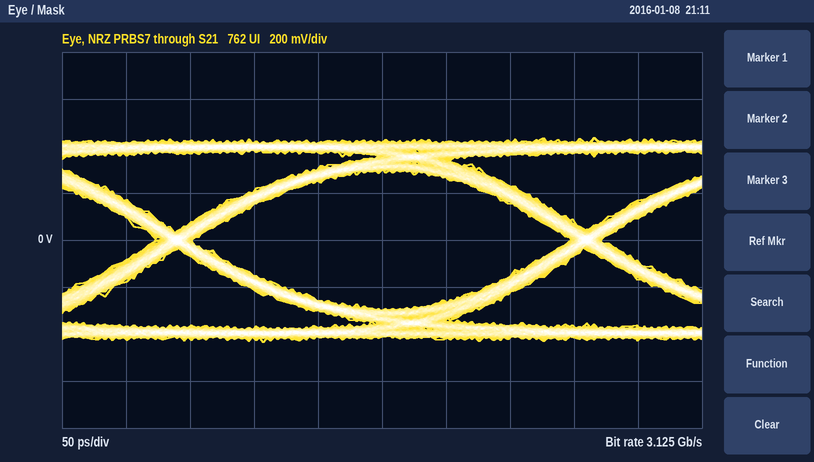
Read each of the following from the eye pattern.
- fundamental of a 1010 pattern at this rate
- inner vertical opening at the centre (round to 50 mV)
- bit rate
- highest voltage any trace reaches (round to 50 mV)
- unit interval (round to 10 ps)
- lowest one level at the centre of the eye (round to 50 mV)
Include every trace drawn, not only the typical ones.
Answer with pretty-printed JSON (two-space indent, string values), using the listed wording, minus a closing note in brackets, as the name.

{
  "fundamental of a 1010 pattern at this rate": "1.5625 GHz",
  "inner vertical opening at the centre": "600 mV",
  "bit rate": "3.125 Gb/s",
  "highest voltage any trace reaches": "450 mV",
  "unit interval": "320 ps",
  "lowest one level at the centre of the eye": "300 mV"
}
